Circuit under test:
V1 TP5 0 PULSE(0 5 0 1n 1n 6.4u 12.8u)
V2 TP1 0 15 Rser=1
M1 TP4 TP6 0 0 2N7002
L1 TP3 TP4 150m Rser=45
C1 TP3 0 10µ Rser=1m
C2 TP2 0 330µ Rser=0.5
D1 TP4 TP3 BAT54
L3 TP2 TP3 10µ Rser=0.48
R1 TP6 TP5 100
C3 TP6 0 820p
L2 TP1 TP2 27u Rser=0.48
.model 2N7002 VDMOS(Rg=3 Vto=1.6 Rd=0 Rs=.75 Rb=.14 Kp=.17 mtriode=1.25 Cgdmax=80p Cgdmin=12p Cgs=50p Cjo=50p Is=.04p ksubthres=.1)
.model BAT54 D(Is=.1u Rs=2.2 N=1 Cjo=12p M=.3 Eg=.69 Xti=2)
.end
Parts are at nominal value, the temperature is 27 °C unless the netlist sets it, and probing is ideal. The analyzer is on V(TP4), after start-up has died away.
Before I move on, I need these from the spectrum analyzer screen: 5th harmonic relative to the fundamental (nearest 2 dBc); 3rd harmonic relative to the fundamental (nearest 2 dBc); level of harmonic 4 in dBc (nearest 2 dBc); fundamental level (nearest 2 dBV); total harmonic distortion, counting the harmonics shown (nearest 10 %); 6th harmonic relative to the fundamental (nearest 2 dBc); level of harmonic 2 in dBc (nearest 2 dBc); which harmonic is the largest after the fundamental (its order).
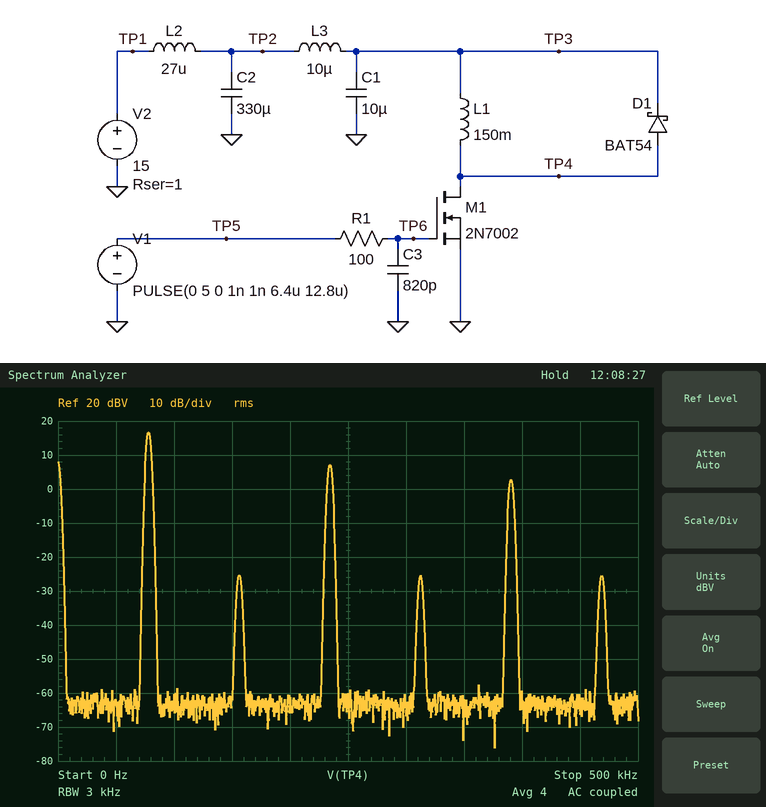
-14 dBc
-10 dBc
-42 dBc
16 dBV
40 %
-42 dBc
-42 dBc
3
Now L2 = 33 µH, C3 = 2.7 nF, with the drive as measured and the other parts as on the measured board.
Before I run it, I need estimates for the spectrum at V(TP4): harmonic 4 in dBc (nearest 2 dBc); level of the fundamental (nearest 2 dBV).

-32 dBc
16 dBV
